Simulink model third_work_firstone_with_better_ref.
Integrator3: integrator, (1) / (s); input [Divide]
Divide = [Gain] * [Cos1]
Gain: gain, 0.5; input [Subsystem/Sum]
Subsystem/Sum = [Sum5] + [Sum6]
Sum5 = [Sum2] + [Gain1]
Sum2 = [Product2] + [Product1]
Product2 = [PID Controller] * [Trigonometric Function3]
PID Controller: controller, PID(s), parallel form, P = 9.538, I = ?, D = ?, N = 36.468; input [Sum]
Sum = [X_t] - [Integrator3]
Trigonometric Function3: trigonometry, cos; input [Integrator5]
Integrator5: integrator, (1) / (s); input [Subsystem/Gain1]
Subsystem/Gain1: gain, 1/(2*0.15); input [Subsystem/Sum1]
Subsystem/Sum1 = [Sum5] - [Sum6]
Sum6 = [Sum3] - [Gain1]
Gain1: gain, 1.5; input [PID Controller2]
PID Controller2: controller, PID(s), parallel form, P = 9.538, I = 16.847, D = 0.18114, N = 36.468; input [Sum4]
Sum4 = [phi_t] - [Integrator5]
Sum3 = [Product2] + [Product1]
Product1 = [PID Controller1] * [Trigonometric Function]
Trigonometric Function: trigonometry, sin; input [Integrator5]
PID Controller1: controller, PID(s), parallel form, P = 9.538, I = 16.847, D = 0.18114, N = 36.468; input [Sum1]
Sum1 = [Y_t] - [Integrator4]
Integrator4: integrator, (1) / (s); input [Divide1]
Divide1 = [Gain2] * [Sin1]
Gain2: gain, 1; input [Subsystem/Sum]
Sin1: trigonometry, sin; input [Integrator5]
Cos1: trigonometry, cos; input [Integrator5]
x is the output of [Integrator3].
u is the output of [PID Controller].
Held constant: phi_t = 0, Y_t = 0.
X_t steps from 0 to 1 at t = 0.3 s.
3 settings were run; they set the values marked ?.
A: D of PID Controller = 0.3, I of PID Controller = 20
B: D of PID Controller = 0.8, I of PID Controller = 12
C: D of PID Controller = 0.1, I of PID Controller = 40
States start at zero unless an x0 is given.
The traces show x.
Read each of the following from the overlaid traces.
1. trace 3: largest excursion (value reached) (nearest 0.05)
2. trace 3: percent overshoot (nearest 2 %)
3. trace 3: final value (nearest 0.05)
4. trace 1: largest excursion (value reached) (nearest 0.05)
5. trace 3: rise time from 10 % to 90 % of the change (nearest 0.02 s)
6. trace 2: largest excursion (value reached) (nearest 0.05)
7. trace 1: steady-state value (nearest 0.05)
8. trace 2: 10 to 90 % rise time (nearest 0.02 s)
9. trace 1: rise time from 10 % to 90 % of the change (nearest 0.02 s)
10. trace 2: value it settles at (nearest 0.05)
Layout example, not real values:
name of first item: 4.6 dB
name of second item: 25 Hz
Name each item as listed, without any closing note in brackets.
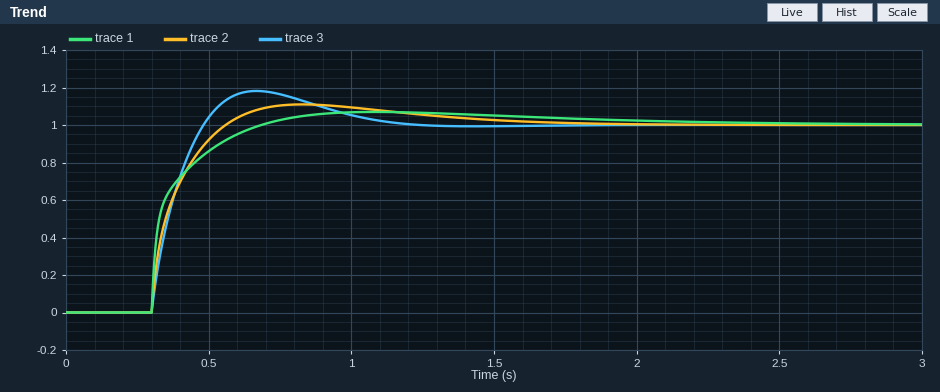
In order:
trace 3: largest excursion (value reached): 1.20
trace 3: percent overshoot: 18 %
trace 3: final value: 1.00
trace 1: largest excursion (value reached): 1.05
trace 3: rise time from 10 % to 90 % of the change: 0.14 s
trace 2: largest excursion (value reached): 1.10
trace 1: steady-state value: 1.00
trace 2: 10 to 90 % rise time: 0.18 s
trace 1: rise time from 10 % to 90 % of the change: 0.24 s
trace 2: value it settles at: 1.00
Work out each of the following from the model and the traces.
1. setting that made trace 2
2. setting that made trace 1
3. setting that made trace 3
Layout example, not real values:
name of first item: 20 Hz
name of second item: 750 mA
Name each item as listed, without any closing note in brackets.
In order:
setting that made trace 2: A
setting that made trace 1: B
setting that made trace 3: C
